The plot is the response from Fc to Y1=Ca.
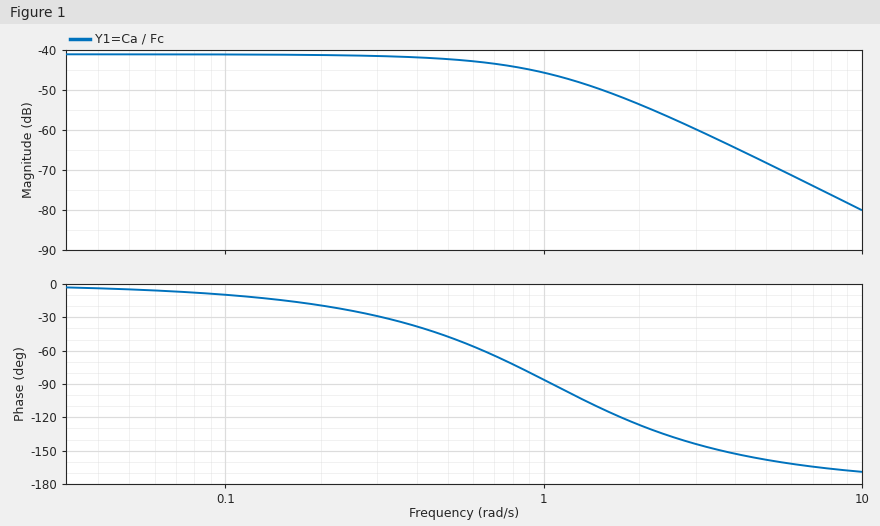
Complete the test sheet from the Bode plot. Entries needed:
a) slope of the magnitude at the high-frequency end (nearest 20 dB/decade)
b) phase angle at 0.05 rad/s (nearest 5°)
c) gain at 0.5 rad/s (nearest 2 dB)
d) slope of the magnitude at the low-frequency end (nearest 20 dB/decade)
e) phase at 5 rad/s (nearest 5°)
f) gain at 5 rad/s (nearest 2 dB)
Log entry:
-40 dB/decade
-5°
-42 dB
0 dB/decade
-160°
-68 dB
